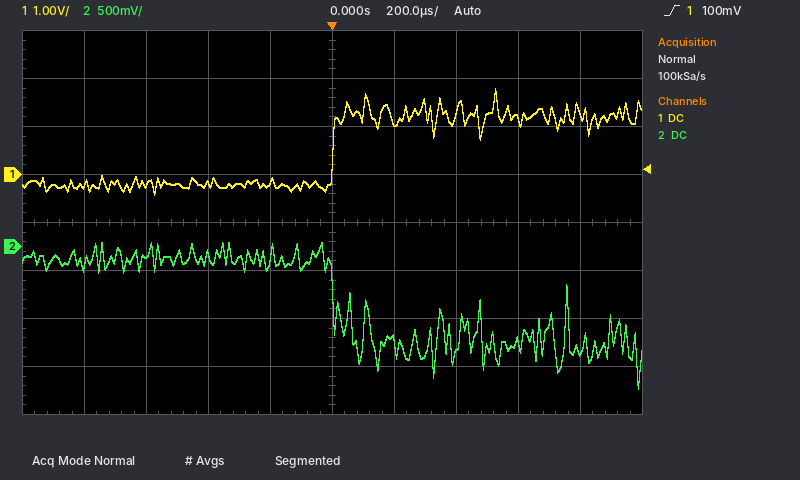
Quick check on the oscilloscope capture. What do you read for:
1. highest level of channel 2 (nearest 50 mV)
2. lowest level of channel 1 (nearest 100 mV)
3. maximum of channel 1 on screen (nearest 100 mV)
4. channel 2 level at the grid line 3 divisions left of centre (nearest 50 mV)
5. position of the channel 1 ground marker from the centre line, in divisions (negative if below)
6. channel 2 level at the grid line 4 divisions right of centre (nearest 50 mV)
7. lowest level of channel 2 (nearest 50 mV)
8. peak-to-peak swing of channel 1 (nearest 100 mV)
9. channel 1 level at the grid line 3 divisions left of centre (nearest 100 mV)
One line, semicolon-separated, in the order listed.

50 mV; -400 mV; 1.8 V; -100 mV; +1.0 div; -1.10 V; -1.50 V; 2.2 V; -200 mV
